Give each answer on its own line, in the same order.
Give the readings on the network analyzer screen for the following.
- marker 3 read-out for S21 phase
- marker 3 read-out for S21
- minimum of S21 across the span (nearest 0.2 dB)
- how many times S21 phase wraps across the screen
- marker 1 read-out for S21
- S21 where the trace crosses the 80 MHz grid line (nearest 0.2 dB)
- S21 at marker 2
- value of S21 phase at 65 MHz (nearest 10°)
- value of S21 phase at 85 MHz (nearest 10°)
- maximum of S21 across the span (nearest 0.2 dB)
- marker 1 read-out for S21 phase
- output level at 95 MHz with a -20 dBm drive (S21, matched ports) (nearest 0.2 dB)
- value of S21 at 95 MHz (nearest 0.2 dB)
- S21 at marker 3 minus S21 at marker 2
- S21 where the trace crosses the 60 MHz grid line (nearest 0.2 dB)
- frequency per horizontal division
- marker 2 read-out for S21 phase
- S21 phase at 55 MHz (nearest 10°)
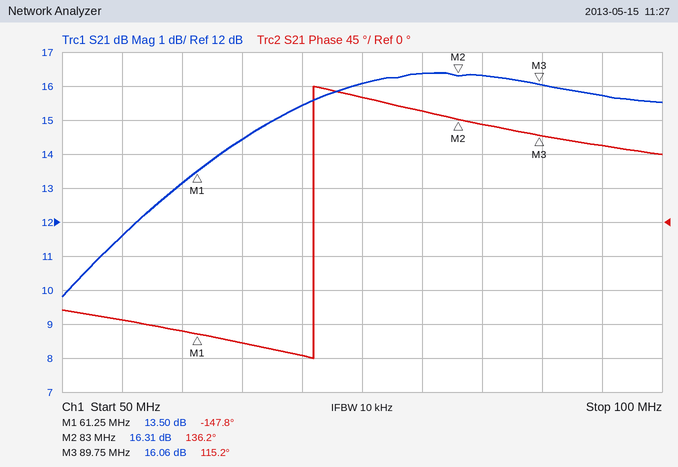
115.2°
16.06 dB
9.8 dB
1
13.50 dB
16.4 dB
16.31 dB
-160°
130°
16.4 dB
-147.8°
-4.2 dBm
15.8 dB
-0.25 dB
13.2 dB
5 MHz
136.2°
-130°
